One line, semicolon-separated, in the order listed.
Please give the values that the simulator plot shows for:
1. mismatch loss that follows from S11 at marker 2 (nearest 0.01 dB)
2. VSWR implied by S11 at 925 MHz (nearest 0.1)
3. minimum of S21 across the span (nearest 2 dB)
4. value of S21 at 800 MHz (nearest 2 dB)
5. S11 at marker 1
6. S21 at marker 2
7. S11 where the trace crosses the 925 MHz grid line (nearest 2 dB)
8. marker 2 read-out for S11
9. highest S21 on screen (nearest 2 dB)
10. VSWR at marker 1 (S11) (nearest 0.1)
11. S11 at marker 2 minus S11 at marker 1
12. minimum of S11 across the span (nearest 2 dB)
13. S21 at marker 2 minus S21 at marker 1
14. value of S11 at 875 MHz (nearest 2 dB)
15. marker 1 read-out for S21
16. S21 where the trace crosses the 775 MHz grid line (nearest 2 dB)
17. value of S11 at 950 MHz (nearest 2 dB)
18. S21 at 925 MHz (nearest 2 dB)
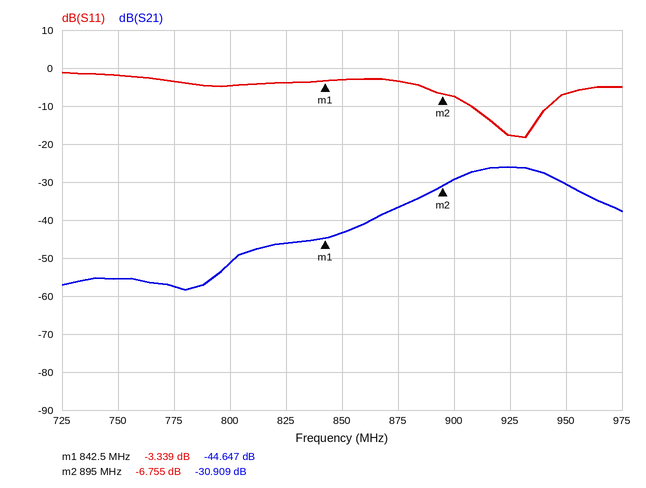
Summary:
1.03 dB; 1.3; -58 dB; -52 dB; -3.339 dB; -30.909 dB; -18 dB; -6.755 dB; -26 dB; 5.3; -3.416 dB; -18 dB; 13.738 dB; -4 dB; -44.647 dB; -58 dB; -6 dB; -26 dB
